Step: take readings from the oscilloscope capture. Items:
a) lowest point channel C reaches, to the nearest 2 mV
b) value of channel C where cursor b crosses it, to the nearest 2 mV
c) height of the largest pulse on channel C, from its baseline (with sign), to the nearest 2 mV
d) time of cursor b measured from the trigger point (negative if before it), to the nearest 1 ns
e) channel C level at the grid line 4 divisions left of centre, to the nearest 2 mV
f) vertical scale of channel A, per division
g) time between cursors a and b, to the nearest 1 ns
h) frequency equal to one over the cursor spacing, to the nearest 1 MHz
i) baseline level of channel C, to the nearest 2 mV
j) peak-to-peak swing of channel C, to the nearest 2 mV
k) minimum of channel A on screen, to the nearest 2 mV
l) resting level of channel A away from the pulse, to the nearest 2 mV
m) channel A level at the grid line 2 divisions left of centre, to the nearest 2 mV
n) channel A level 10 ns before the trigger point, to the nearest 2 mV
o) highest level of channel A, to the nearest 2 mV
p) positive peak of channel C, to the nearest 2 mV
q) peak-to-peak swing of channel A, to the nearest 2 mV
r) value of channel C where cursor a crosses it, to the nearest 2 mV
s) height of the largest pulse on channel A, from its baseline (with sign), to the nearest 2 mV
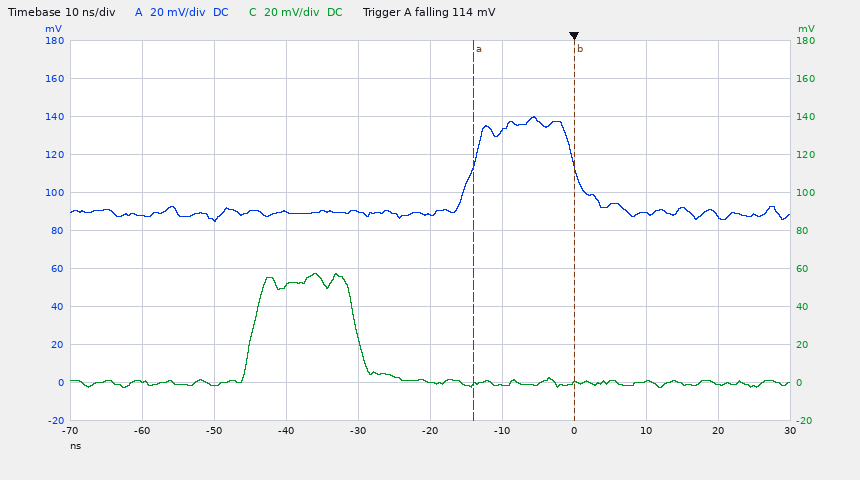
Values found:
-2 mV
0 mV
+58 mV
0 ns
0 mV
20 mV
14 ns
71 MHz
0 mV
60 mV
84 mV
90 mV
90 mV
132 mV
140 mV
58 mV
56 mV
-2 mV
+50 mV
